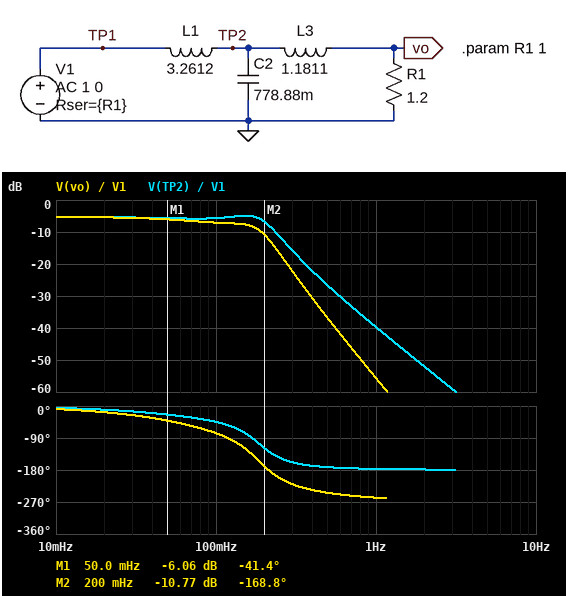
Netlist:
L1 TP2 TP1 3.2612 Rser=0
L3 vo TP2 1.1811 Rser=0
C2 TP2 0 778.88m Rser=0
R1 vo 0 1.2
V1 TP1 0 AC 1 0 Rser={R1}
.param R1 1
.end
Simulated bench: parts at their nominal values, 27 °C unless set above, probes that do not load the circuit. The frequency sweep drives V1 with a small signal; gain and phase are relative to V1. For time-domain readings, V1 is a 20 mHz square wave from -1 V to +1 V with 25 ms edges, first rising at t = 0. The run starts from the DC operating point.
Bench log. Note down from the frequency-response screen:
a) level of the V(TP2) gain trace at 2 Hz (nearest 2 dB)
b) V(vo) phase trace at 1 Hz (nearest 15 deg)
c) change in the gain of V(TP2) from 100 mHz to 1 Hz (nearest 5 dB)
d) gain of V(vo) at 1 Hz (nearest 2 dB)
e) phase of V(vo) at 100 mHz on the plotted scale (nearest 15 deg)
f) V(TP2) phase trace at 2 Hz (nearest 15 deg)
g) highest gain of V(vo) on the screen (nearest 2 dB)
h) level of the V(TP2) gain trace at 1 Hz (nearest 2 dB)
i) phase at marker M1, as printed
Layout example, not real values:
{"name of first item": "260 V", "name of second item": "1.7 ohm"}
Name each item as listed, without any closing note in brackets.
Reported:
{"level of the V(TP2) gain trace at 2 Hz": "-52 dB", "V(vo) phase trace at 1 Hz": "-255 deg", "change in the gain of V(TP2) from 100 mHz to 1 Hz": "-35 dB", "gain of V(vo) at 1 Hz": "-56 dB", "phase of V(vo) at 100 mHz on the plotted scale": "-75 deg", "V(TP2) phase trace at 2 Hz": "-180 deg", "highest gain of V(vo) on the screen": "-6 dB", "level of the V(TP2) gain trace at 1 Hz": "-40 dB", "phase at marker M1, as printed": "-41.4 deg"}
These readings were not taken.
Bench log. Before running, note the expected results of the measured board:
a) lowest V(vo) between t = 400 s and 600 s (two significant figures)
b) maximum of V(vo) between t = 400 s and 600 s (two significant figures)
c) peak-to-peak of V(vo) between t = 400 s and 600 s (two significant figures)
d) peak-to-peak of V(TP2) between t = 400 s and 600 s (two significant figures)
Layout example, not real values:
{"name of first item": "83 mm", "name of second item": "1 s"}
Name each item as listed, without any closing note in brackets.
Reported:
{"lowest V(vo) between t = 400 s and 600 s": "-550 mV", "maximum of V(vo) between t = 400 s and 600 s": "550 mV", "peak-to-peak of V(vo) between t = 400 s and 600 s": "1.1 V", "peak-to-peak of V(TP2) between t = 400 s and 600 s": "1.3 V"}
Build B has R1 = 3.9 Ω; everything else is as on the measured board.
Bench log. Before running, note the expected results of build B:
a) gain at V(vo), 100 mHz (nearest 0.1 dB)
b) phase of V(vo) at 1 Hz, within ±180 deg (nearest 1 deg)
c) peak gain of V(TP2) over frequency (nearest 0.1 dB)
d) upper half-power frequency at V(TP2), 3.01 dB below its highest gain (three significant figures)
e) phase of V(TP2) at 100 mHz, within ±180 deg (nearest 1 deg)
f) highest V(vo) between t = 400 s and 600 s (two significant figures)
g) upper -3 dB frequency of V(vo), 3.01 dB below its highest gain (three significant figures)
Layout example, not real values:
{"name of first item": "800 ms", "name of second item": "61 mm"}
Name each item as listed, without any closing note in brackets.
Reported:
{"gain at V(vo), 100 mHz": "-0.2 dB", "phase of V(vo) at 1 Hz, within ±180 deg": "121 deg", "peak gain of V(TP2) over frequency": "0 dB", "upper half-power frequency at V(TP2), 3.01 dB below its highest gain": "140 mHz", "phase of V(TP2) at 100 mHz, within ±180 deg": "-70 deg", "highest V(vo) between t = 400 s and 600 s": "1.1 V", "upper -3 dB frequency of V(vo), 3.01 dB below its highest gain": "138 mHz"}
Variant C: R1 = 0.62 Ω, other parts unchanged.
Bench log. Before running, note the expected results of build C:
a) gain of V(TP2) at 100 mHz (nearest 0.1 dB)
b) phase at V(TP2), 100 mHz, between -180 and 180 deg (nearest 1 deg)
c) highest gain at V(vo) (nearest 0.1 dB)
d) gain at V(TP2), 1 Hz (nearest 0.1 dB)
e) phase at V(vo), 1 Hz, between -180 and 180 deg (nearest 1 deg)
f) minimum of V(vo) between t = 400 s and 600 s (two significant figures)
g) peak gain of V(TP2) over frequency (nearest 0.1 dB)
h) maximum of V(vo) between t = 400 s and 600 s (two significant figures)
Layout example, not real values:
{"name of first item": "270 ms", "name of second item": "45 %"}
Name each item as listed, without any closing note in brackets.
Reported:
{"gain of V(TP2) at 100 mHz": "-8.0 dB", "phase at V(TP2), 100 mHz, between -180 and 180 deg": "-25 deg", "highest gain at V(vo)": "-8.3 dB", "gain at V(TP2), 1 Hz": "-39.7 dB", "phase at V(vo), 1 Hz, between -180 and 180 deg": "98 deg", "minimum of V(vo) between t = 400 s and 600 s": "-390 mV", "peak gain of V(TP2) over frequency": "-2.6 dB", "maximum of V(vo) between t = 400 s and 600 s": "390 mV"}
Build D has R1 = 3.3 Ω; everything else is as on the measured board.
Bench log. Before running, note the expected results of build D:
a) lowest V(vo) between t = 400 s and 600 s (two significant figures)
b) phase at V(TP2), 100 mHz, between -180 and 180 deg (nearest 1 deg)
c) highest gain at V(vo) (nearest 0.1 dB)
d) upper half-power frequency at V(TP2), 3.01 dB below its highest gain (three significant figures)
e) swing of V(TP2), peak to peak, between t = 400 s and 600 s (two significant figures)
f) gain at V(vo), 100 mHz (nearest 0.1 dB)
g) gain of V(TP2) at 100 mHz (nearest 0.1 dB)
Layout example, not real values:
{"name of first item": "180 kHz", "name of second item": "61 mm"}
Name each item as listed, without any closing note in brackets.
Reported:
{"lowest V(vo) between t = 400 s and 600 s": "-1.0 V", "phase at V(TP2), 100 mHz, between -180 and 180 deg": "-68 deg", "highest gain at V(vo)": "-0.9 dB", "upper half-power frequency at V(TP2), 3.01 dB below its highest gain": "145 mHz", "swing of V(TP2), peak to peak, between t = 400 s and 600 s": "2.1 V", "gain at V(vo), 100 mHz": "-1.0 dB", "gain of V(TP2) at 100 mHz": "-0.8 dB"}
